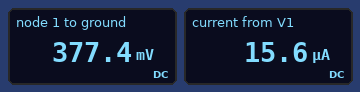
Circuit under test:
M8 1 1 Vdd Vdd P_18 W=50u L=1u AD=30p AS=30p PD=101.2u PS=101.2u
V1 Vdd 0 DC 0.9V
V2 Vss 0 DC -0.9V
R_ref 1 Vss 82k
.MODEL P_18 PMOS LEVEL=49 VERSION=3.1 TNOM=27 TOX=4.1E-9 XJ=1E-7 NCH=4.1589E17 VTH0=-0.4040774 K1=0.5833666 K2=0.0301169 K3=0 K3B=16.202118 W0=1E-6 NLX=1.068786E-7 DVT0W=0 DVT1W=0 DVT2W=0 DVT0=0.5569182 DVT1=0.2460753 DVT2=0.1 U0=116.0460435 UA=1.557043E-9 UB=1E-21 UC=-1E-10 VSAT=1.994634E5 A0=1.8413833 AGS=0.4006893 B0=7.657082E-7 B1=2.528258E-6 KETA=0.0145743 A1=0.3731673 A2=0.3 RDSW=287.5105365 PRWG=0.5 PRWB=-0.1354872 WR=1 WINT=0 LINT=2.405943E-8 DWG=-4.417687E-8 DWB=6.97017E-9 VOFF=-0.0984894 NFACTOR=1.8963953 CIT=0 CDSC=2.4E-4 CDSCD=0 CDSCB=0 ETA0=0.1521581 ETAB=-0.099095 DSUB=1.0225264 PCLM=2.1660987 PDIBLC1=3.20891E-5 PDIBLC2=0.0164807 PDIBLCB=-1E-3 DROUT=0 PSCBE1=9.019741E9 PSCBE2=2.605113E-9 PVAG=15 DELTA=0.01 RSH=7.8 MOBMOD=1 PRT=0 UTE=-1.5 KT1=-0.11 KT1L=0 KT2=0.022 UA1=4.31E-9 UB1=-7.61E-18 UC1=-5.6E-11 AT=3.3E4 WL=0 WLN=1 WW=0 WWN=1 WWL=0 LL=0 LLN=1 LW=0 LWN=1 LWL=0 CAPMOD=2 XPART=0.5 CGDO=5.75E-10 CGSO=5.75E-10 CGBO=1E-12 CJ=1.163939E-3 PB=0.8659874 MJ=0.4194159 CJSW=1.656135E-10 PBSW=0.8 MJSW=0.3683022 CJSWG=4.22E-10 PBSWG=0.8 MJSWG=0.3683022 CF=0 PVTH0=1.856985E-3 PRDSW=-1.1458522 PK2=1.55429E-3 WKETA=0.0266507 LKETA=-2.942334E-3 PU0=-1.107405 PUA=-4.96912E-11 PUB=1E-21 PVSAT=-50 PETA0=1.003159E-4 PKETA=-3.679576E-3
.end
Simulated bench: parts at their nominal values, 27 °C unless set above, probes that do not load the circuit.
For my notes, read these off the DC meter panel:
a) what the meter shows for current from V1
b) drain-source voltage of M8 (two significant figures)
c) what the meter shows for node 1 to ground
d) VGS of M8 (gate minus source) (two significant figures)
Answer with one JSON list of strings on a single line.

["15.6 µA", "-520 mV", "377.4 mV", "-520 mV"]
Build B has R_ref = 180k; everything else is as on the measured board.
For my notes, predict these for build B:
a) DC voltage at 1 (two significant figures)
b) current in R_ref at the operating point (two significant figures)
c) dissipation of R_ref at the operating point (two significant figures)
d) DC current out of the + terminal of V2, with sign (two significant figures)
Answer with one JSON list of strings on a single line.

["420 mV", "7.3 µA", "9.7 µW", "-7.3 µA"]
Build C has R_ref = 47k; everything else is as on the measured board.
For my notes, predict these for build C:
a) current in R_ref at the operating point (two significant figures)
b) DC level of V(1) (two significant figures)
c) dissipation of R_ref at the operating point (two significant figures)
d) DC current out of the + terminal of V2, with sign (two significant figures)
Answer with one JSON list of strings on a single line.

["26 µA", "340 mV", "33 µW", "-26 µA"]
